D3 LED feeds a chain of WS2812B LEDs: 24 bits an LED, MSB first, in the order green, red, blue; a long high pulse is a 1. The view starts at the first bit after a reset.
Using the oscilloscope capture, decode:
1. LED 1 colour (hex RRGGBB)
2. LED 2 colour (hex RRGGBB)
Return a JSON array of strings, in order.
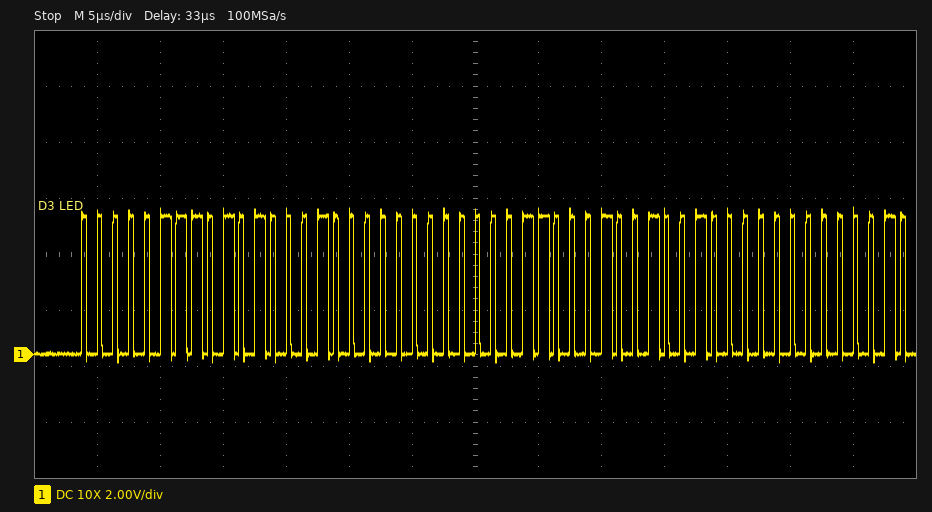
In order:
["#510700", "#490C00"]
